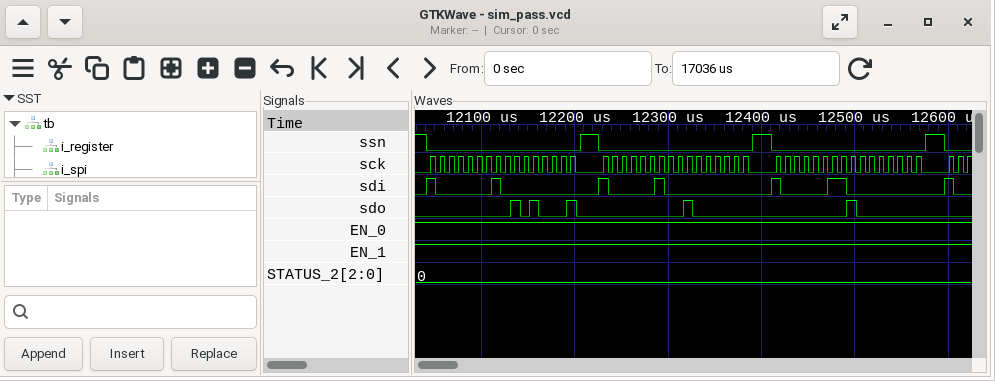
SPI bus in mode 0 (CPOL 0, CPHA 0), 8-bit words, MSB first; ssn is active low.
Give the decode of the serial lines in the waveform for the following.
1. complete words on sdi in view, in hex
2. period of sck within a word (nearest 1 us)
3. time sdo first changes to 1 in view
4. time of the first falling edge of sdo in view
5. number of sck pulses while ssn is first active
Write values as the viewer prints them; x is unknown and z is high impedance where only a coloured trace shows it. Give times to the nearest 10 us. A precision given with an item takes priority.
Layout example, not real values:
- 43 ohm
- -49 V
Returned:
- 81, 00, 82, 00, 83, 00
- 10 us
- 12130 us
- 12140 us
- 16
